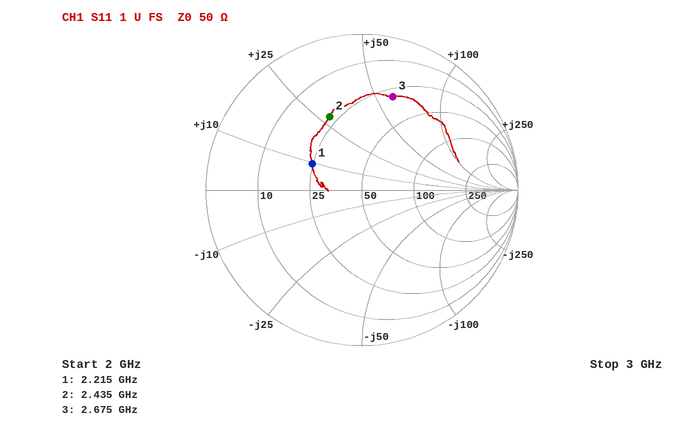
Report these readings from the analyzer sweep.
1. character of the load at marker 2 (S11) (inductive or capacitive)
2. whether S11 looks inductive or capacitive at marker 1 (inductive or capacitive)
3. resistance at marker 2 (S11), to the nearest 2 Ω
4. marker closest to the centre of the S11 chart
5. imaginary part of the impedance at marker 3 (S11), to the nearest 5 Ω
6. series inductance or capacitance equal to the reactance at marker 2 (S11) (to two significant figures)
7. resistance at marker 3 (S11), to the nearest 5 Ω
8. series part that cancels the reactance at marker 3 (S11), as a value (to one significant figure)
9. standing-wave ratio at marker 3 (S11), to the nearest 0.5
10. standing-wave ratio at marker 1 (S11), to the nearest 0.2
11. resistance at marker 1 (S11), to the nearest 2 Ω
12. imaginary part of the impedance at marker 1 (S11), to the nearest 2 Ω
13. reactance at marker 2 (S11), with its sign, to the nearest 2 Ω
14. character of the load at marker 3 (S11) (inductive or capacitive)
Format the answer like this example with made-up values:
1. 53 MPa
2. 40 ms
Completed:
1. inductive
2. inductive
3. 22 Ω
4. marker 1
5. +60 Ω
6. 1.8 nH
7. 30 Ω
8. 1.0 pF
9. 4.5
10. 2.2
11. 24 Ω
12. +10 Ω
13. +28 Ω
14. inductive
